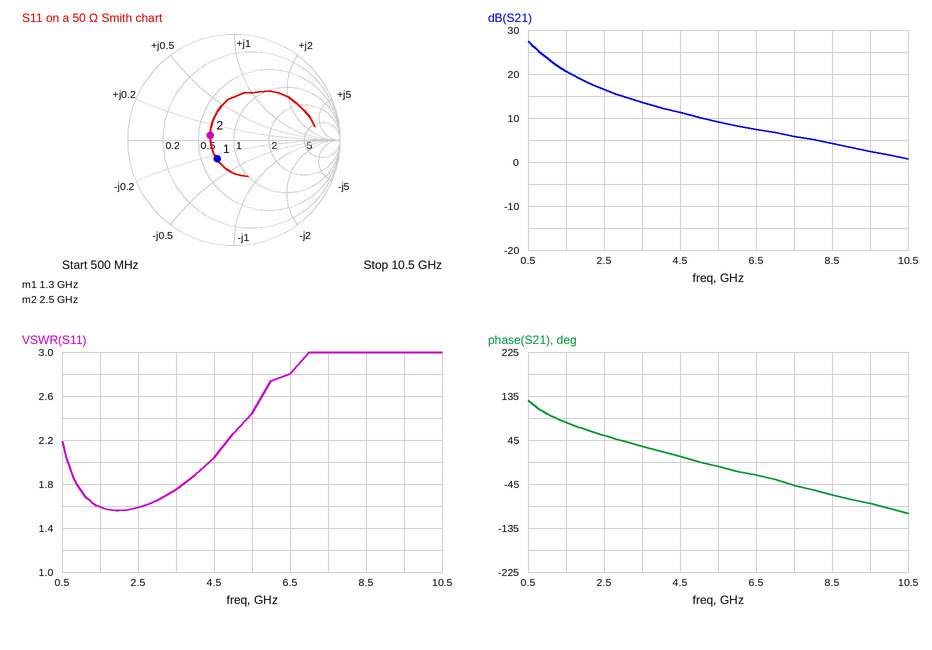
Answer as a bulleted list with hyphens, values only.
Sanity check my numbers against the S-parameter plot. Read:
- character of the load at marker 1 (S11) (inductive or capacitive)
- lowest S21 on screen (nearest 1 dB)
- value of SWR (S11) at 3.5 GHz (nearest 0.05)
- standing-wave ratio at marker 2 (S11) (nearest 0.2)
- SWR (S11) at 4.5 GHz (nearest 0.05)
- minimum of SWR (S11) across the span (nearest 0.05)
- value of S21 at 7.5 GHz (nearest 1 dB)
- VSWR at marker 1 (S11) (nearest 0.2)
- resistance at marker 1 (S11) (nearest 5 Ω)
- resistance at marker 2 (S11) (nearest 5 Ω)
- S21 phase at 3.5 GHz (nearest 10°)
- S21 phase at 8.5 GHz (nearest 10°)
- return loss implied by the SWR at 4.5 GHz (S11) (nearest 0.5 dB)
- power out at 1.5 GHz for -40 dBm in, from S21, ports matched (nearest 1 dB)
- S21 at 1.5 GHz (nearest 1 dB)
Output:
- capacitive
- 1 dB
- 1.75
- 1.6
- 2.05
- 1.55
- 6 dB
- 1.6
- 35 Ω
- 30 Ω
- 30°
- -70°
- 9.5 dB
- -19 dBm
- 21 dB
